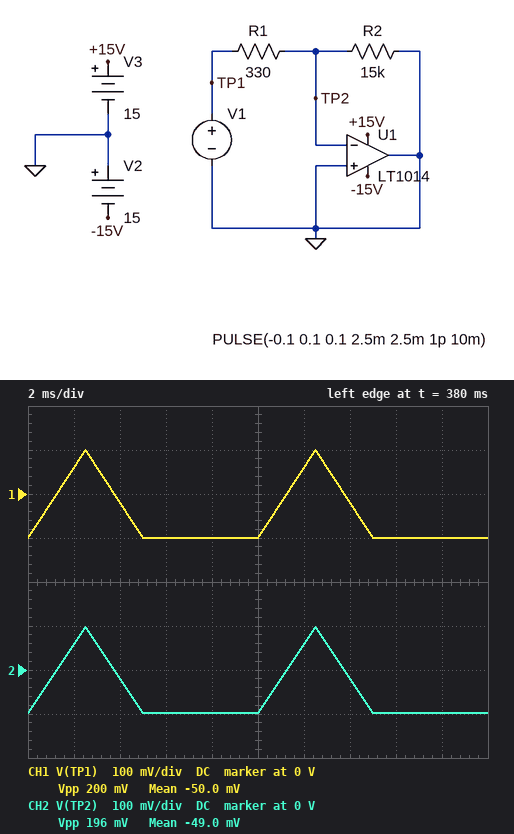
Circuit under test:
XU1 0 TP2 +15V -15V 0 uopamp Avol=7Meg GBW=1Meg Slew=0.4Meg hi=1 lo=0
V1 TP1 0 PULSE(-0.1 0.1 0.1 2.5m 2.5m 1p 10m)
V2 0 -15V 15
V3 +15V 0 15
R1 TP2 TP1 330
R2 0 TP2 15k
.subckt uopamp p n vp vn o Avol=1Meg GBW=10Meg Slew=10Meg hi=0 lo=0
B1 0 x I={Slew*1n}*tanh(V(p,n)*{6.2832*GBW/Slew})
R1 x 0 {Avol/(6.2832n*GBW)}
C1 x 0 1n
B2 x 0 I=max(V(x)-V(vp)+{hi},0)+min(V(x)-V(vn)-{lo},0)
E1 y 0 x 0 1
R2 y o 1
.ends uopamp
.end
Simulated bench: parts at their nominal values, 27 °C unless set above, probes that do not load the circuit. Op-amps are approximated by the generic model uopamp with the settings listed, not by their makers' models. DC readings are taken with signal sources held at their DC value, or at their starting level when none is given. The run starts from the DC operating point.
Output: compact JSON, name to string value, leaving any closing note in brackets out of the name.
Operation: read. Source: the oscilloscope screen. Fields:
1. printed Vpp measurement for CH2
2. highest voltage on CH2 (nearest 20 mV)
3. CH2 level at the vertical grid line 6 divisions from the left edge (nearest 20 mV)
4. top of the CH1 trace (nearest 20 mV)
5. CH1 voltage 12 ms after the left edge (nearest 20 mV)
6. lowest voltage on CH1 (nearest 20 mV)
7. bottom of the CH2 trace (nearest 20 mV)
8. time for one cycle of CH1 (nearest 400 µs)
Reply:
{"printed Vpp measurement for CH2": "196 mV", "highest voltage on CH2": "100 mV", "CH2 level at the vertical grid line 6 divisions from the left edge": "60 mV", "top of the CH1 trace": "100 mV", "CH1 voltage 12 ms after the left edge": "60 mV", "lowest voltage on CH1": "-100 mV", "bottom of the CH2 trace": "-100 mV", "time for one cycle of CH1": "10.0 ms"}
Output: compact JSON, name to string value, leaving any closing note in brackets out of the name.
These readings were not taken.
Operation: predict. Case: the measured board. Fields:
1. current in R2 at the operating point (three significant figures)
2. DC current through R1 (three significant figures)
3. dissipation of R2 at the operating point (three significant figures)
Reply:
{"current in R2 at the operating point": "6.52 µA", "DC current through R1": "6.52 µA", "dissipation of R2 at the operating point": "638 nW"}
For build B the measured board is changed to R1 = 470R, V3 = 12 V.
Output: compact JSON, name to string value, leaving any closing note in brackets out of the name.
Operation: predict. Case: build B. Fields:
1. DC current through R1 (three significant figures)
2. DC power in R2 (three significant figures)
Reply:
{"DC current through R1": "6.46 µA", "DC power in R2": "627 nW"}
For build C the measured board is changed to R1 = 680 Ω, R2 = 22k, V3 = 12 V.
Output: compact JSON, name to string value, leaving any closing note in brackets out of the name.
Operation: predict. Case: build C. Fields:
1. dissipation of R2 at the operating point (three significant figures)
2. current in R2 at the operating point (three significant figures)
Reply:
{"dissipation of R2 at the operating point": "428 nW", "current in R2 at the operating point": "4.41 µA"}
